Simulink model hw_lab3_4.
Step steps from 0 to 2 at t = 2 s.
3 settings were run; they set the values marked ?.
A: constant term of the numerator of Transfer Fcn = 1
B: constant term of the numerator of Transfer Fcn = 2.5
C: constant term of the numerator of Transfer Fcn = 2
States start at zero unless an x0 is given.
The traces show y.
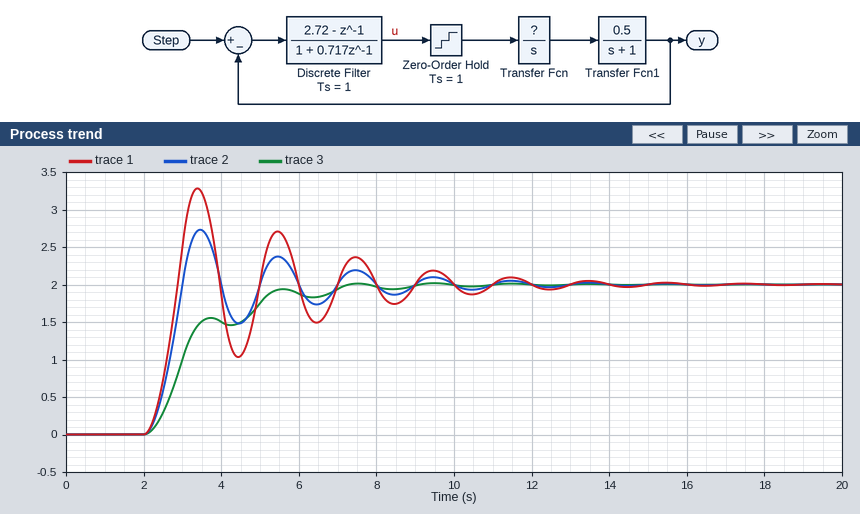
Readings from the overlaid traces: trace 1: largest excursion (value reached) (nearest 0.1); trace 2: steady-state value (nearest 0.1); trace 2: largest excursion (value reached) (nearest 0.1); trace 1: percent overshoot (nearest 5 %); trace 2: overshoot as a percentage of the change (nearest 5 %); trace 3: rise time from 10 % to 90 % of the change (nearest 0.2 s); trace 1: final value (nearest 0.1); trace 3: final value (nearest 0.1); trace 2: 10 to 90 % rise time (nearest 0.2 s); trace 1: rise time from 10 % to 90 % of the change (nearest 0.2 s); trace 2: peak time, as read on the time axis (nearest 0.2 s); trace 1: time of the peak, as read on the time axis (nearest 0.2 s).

3.3
2.0
2.7
65 %
35 %
2.6 s
2.0
2.0
0.6 s
0.6 s
3.4 s
3.4 s
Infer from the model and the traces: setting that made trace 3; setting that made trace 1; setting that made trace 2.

A
B
C
